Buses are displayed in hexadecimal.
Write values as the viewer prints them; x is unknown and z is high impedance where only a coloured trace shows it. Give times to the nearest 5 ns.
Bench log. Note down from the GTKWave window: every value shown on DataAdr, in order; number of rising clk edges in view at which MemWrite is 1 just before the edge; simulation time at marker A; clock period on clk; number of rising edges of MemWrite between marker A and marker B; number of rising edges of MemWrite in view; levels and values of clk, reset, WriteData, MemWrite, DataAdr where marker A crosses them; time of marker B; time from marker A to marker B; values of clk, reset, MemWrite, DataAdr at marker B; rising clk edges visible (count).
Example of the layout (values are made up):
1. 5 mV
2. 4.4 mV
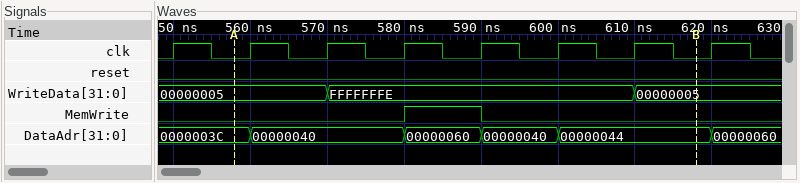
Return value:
1. 0000003C, 00000040, 00000060, 00000040, 00000044, 00000060
2. 1
3. 560 ns
4. 10 ns
5. 1
6. 1
7. clk=0, reset=0, WriteData=00000005, MemWrite=0, DataAdr=0000003C
8. 620 ns
9. 60 ns
10. clk=0, reset=0, MemWrite=0, DataAdr=00000044
11. 8
